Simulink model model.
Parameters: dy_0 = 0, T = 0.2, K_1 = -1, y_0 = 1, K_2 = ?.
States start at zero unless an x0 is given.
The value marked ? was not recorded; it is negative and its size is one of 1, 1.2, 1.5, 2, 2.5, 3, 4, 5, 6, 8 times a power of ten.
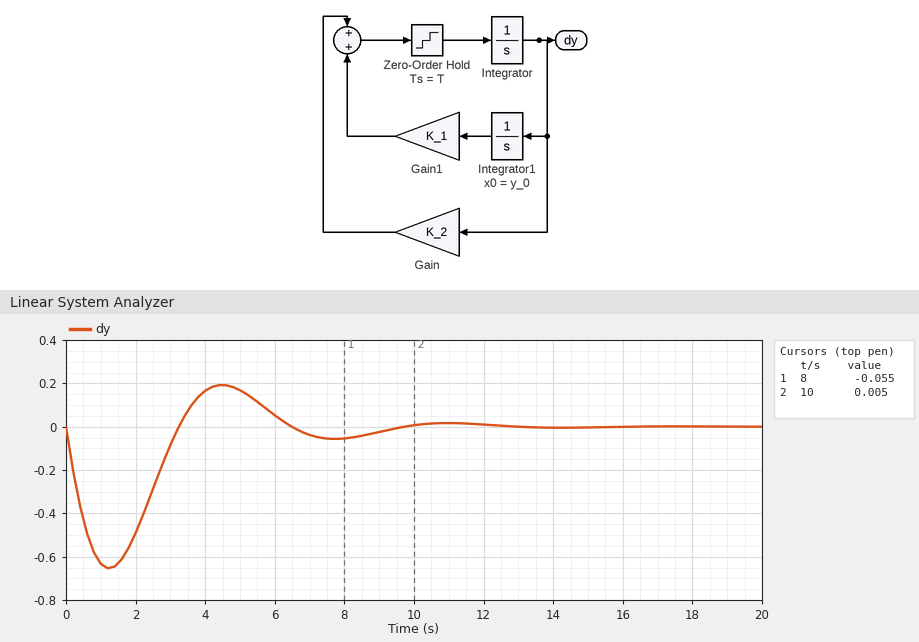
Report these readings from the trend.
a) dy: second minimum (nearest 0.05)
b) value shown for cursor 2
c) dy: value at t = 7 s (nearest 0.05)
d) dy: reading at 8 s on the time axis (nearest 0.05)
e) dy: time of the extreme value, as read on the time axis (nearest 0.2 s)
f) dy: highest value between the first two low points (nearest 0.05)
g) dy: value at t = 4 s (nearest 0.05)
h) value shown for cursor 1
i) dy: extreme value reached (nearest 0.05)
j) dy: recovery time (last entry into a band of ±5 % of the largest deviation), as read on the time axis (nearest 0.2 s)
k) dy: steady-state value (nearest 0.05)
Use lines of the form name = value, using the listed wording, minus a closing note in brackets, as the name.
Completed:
dy: second minimum = -0.05
value shown for cursor 2 = 0.005
dy: value at t = 7 s = -0.05
dy: reading at 8 s on the time axis = -0.05
dy: time of the extreme value, as read on the time axis = 1.2 s
dy: highest value between the first two low points = 0.20
dy: value at t = 4 s = 0.15
value shown for cursor 1 = -0.055
dy: extreme value reached = -0.65
dy: recovery time (last entry into a band of ±5 % of the largest deviation), as read on the time axis = 8.8 s
dy: steady-state value = 0.00
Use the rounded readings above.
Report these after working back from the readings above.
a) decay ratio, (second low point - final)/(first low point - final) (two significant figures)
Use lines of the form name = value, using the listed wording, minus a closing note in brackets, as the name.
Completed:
decay ratio, (second low point - final)/(first low point - final) = 0.077
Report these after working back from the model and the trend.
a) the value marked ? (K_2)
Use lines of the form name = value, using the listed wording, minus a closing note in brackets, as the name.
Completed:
the value marked ? = -0.8
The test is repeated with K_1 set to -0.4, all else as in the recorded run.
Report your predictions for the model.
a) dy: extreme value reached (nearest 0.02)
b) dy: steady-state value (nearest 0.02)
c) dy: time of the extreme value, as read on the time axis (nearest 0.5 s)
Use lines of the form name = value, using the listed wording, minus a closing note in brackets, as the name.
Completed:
dy: extreme value reached = -0.32
dy: steady-state value = 0.00
dy: time of the extreme value, as read on the time axis = 2.0 s
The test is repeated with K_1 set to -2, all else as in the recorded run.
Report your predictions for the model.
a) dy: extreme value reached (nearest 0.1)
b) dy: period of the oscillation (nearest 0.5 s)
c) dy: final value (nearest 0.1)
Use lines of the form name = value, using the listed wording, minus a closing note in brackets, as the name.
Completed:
dy: extreme value reached = -1.1
dy: period of the oscillation = 4.5 s
dy: final value = 0.0
